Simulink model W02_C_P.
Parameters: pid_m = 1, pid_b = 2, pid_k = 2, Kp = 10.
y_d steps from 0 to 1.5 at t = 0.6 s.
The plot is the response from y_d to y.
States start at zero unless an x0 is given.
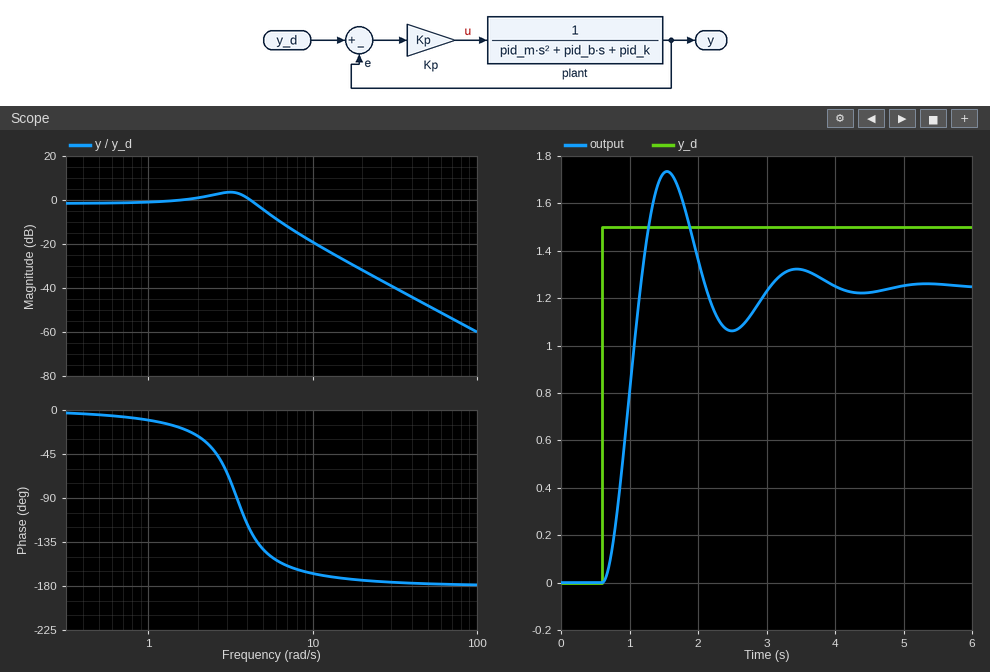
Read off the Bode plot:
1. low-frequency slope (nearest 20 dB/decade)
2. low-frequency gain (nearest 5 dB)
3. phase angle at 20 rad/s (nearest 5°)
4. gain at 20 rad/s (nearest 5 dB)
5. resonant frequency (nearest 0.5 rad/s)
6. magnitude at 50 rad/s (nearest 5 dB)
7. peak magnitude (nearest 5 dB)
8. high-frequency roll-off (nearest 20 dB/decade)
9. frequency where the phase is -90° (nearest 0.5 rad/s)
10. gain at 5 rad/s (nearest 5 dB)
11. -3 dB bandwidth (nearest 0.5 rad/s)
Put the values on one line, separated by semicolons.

0 dB/decade; 0 dB; -175°; -30 dB; 3.0 rad/s; -50 dB; 5 dB; -40 dB/decade; 3.5 rad/s; -5 dB; 5.0 rad/s
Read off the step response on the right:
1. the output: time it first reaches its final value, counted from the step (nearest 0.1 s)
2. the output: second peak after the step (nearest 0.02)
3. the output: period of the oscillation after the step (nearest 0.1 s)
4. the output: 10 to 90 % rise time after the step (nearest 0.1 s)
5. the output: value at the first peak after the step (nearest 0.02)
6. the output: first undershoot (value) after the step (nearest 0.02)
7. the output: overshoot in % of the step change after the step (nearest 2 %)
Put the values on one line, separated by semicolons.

0.6 s; 1.32; 1.9 s; 0.4 s; 1.74; 1.06; 38 %
